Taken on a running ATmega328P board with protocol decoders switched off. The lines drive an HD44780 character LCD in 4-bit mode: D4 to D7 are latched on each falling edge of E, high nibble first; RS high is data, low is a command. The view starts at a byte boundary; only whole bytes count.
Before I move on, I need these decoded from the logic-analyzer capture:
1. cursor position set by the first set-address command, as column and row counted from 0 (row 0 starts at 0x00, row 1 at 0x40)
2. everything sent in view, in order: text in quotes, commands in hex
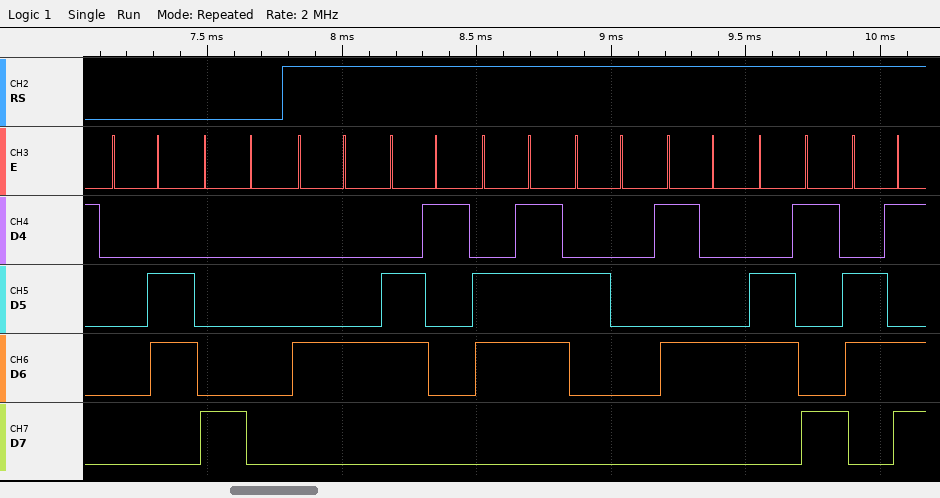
column 0, row 0
0x06 0x80 "Dag Tim"
